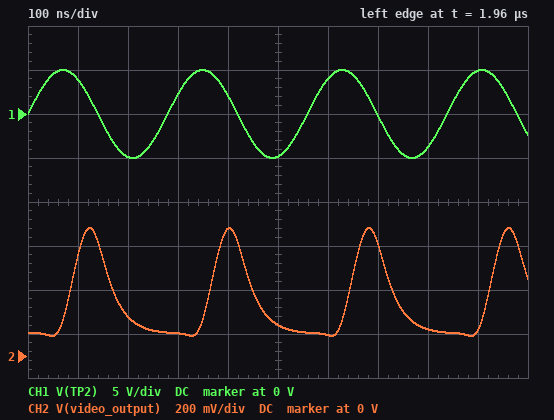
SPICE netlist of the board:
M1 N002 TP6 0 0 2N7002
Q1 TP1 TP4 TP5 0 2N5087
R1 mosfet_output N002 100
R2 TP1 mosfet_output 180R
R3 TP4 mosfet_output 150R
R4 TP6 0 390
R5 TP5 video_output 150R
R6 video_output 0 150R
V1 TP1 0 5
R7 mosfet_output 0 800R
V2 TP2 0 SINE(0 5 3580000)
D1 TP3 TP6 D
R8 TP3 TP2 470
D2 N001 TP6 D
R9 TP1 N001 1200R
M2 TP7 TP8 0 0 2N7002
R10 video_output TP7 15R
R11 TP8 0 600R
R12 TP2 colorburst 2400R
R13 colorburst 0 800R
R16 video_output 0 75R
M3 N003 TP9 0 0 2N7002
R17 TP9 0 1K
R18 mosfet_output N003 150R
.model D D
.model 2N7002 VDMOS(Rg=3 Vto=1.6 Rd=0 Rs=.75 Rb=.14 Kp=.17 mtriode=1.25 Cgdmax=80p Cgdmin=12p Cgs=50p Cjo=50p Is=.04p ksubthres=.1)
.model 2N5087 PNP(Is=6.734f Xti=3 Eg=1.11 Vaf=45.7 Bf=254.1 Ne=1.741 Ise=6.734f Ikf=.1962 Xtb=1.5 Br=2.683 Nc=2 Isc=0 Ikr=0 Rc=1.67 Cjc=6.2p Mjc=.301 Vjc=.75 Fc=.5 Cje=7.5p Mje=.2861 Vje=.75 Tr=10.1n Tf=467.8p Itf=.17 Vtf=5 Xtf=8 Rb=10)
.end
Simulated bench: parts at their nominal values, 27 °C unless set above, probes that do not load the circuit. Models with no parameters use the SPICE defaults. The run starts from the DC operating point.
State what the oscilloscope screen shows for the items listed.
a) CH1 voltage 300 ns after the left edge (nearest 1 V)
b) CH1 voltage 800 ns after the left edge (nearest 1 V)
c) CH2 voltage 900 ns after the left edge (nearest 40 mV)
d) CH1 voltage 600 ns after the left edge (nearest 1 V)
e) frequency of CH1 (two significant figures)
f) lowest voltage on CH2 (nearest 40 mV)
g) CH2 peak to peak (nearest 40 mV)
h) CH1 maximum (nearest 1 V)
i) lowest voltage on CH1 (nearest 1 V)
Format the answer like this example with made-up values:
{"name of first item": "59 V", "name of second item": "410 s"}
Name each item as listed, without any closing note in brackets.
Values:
{"CH1 voltage 300 ns after the left edge": "2 V", "CH1 voltage 800 ns after the left edge": "-4 V", "CH2 voltage 900 ns after the left edge": "120 mV", "CH1 voltage 600 ns after the left edge": "4 V", "frequency of CH1": "3.6 MHz", "lowest voltage on CH2": "80 mV", "CH2 peak to peak": "480 mV", "CH1 maximum": "5 V", "lowest voltage on CH1": "-5 V"}
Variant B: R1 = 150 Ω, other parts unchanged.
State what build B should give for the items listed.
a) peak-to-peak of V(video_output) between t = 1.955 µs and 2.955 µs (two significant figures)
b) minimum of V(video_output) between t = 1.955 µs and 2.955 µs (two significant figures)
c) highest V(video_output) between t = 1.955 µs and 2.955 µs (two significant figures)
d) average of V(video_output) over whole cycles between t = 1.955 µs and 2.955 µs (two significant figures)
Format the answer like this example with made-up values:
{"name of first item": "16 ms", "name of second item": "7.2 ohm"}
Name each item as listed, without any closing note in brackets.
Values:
{"peak-to-peak of V(video_output) between t = 1.955 µs and 2.955 µs": "420 mV", "minimum of V(video_output) between t = 1.955 µs and 2.955 µs": "92 mV", "highest V(video_output) between t = 1.955 µs and 2.955 µs": "510 mV", "average of V(video_output) over whole cycles between t = 1.955 µs and 2.955 µs": "230 mV"}
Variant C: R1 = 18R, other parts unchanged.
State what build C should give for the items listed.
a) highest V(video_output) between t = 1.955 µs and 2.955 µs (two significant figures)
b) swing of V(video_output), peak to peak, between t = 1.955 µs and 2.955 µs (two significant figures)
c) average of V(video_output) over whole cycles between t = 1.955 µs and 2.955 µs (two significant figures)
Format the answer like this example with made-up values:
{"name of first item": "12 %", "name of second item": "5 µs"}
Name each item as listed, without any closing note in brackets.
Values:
{"highest V(video_output) between t = 1.955 µs and 2.955 µs": "770 mV", "swing of V(video_output), peak to peak, between t = 1.955 µs and 2.955 µs": "680 mV", "average of V(video_output) over whole cycles between t = 1.955 µs and 2.955 µs": "280 mV"}
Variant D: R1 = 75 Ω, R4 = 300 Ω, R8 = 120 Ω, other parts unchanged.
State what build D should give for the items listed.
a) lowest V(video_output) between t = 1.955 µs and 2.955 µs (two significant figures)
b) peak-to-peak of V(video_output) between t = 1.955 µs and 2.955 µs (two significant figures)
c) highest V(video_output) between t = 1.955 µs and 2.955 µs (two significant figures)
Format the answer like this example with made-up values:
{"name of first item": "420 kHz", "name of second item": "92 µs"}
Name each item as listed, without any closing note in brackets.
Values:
{"lowest V(video_output) between t = 1.955 µs and 2.955 µs": "98 mV", "peak-to-peak of V(video_output) between t = 1.955 µs and 2.955 µs": "1.1 V", "highest V(video_output) between t = 1.955 µs and 2.955 µs": "1.2 V"}
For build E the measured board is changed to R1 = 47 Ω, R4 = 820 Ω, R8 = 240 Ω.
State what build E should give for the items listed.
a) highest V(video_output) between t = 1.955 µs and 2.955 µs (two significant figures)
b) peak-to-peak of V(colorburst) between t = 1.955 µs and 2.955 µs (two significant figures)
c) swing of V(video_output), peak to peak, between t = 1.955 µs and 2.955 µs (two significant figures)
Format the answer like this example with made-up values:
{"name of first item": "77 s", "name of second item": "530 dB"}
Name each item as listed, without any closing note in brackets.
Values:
{"highest V(video_output) between t = 1.955 µs and 2.955 µs": "1.2 V", "peak-to-peak of V(colorburst) between t = 1.955 µs and 2.955 µs": "2.5 V", "swing of V(video_output), peak to peak, between t = 1.955 µs and 2.955 µs": "4.2 mV"}
